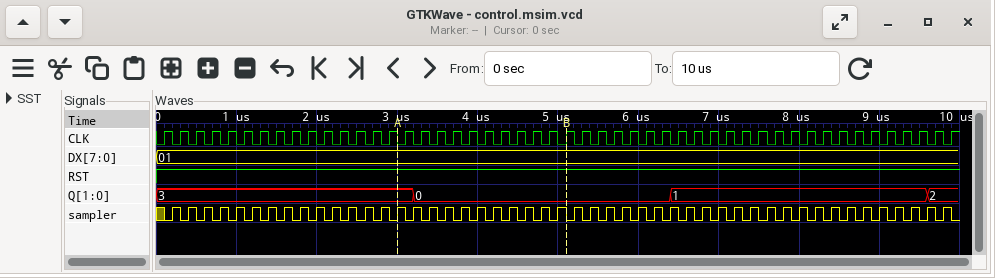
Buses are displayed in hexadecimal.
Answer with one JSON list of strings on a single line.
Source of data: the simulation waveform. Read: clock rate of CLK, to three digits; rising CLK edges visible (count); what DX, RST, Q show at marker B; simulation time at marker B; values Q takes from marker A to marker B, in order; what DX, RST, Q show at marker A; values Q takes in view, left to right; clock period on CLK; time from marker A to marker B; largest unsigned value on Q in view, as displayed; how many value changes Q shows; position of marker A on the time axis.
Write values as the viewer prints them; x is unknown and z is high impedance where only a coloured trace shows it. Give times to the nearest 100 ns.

["5.00 MHz", "50", "DX=01, RST=1, Q=0", "5100 ns", "3, 0", "DX=01, RST=1, Q=3", "3, 0, 1, 2", "200 ns", "2100 ns", "3", "3", "3000 ns"]
